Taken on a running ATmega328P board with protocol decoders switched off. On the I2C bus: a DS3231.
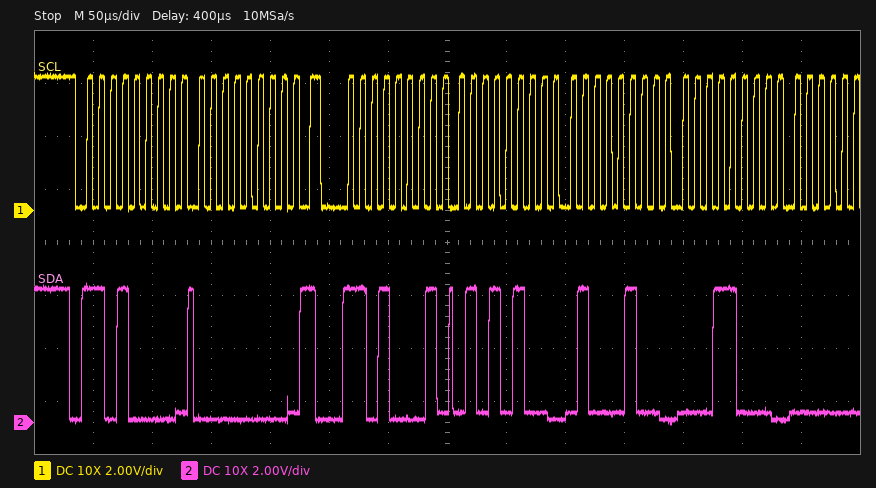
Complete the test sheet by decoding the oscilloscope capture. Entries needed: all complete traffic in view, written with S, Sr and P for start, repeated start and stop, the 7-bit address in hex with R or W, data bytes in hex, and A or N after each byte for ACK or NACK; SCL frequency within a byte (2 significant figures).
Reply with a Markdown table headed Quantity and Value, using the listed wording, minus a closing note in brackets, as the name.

| Quantity | Value |
|---|---|
| all complete traffic in view, written with S, Sr and P for start, repeated start and stop, the 7-bit address in hex with R or W, data bytes in hex, and A or N after each byte for ACK or NACK | S 68W A 00 A Sr 68R A 54 A 44 A 18 A |
| SCL frequency within a byte | 100 kHz |
